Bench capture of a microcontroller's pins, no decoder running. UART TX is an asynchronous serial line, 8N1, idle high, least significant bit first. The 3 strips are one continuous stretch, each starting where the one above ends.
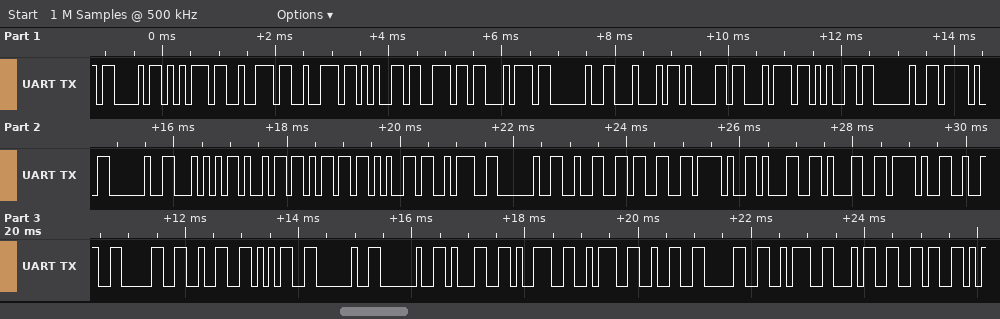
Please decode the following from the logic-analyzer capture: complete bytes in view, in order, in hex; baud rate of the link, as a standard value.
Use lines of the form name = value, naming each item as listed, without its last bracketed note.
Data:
complete bytes in view, in order, in hex = 43 75 72 72 65 6E 74 20 44 61 74 65 20 2F 20 54 69 6D 65 3A 20 32 33 2F 31 31 2F 32 30 32 35 20 20 31 39 3A 32 30 3A 34 36
baud rate of the link, as a standard value = 9600 baud
